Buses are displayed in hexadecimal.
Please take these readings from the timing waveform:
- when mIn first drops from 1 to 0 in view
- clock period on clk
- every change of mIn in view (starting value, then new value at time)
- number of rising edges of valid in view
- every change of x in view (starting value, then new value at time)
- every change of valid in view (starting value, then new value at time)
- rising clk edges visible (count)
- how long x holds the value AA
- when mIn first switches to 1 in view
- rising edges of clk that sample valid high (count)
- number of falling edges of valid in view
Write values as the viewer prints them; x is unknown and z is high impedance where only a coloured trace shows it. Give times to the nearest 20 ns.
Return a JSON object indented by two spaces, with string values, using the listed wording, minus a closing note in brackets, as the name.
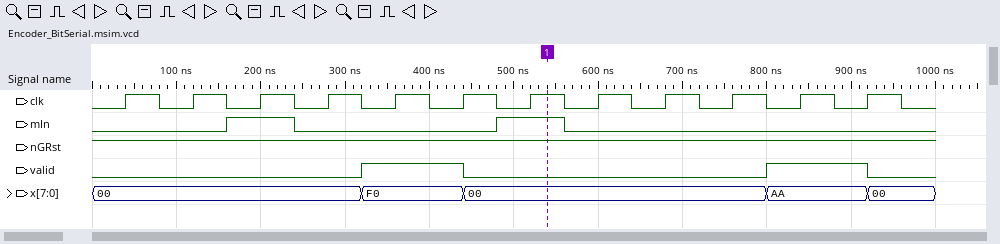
{
  "when mIn first drops from 1 to 0 in view": "240 ns",
  "clock period on clk": "80 ns",
  "every change of mIn in view": "0, 1 at 160 ns, 0 at 240 ns, 1 at 480 ns, 0 at 560 ns",
  "number of rising edges of valid in view": "2",
  "every change of x in view": "00, F0 at 320 ns, 00 at 440 ns, AA at 800 ns, 00 at 920 ns",
  "every change of valid in view": "0, 1 at 320 ns, 0 at 440 ns, 1 at 800 ns, 0 at 920 ns",
  "rising clk edges visible": "12",
  "how long x holds the value AA": "120 ns",
  "when mIn first switches to 1 in view": "160 ns",
  "rising edges of clk that sample valid high": "4",
  "number of falling edges of valid in view": "2"
}
